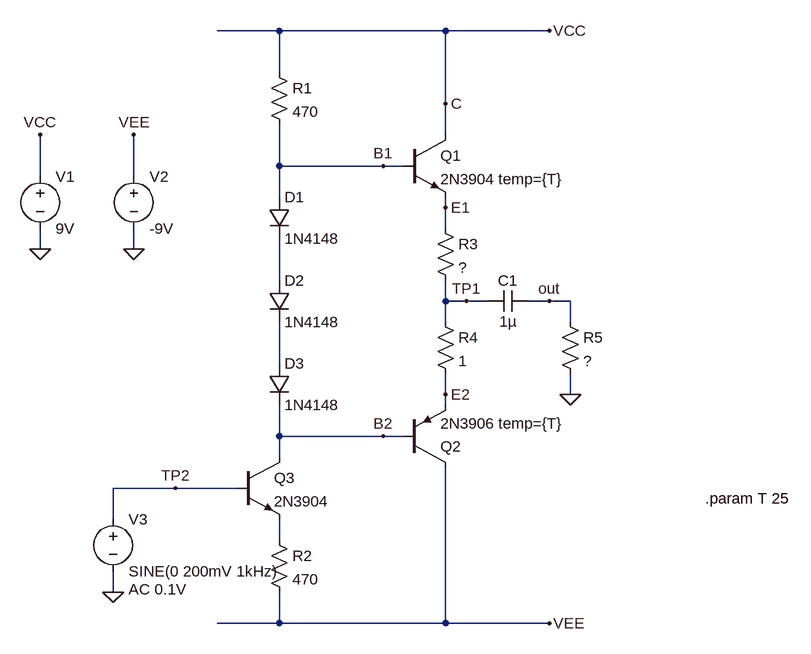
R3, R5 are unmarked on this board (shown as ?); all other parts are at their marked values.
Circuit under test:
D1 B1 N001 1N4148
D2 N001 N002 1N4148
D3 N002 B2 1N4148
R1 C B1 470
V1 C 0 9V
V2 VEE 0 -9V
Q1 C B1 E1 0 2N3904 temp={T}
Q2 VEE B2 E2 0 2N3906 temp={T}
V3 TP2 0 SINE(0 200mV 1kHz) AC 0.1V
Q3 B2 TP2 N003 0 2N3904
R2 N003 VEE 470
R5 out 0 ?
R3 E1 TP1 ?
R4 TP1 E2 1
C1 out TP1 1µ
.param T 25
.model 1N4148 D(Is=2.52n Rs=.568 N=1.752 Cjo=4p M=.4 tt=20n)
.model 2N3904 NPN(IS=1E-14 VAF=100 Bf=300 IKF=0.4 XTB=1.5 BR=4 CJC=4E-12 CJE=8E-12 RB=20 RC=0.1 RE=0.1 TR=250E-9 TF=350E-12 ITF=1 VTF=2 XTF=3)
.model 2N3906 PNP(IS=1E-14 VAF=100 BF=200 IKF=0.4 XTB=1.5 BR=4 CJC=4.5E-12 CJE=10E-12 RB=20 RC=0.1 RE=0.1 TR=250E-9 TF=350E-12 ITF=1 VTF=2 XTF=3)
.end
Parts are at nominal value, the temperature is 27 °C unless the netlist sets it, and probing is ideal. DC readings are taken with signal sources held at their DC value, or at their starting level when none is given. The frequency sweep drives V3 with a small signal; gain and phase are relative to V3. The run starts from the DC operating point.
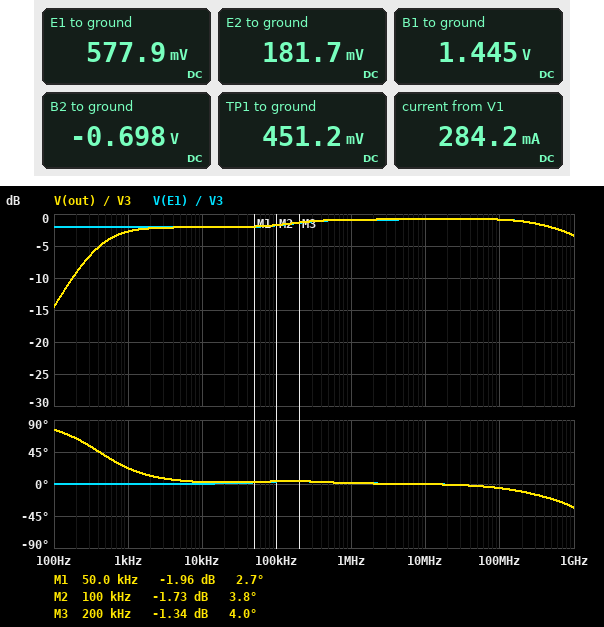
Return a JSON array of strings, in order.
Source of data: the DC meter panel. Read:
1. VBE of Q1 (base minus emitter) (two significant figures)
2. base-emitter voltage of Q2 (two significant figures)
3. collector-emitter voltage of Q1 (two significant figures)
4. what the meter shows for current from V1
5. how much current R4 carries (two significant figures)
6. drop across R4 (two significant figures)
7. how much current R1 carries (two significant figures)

["870 mV", "-880 mV", "8.4 V", "284.2 mA", "270 mA", "270 mV", "16 mA"]
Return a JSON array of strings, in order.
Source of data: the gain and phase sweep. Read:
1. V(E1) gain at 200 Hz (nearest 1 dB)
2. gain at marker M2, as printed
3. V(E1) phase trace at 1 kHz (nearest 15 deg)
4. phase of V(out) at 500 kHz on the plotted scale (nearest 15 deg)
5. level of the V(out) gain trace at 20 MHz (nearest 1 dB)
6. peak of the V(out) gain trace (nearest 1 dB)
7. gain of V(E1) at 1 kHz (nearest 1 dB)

["-2 dB", "-1.73 dB", "0 deg", "0 deg", "-1 dB", "-1 dB", "-2 dB"]
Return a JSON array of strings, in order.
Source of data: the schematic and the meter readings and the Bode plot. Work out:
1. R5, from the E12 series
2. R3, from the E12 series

["390 Ω", "0.47 Ω"]
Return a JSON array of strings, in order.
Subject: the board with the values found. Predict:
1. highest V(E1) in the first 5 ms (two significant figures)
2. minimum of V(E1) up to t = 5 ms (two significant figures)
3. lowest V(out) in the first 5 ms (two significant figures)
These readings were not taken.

["740 mV", "450 mV", "-140 mV"]
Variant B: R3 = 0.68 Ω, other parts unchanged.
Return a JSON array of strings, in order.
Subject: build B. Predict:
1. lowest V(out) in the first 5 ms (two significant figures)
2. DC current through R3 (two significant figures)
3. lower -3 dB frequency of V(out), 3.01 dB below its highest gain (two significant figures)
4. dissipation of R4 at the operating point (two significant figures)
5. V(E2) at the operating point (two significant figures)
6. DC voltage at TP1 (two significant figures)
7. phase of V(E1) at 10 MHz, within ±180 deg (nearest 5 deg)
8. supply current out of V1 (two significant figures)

["-150 mV", "250 mA", "560 Hz", "61 mW", "170 mV", "420 mV", "0 deg", "260 mA"]
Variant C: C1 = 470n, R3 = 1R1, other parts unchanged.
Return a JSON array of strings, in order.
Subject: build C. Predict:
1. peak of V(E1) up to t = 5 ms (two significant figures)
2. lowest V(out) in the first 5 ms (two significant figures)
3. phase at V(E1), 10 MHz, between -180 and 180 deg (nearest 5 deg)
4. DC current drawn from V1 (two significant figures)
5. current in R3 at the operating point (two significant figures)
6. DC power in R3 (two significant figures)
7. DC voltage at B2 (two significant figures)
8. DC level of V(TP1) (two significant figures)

["760 mV", "-120 mV", "0 deg", "230 mA", "210 mA", "50 mW", "-710 mV", "360 mV"]
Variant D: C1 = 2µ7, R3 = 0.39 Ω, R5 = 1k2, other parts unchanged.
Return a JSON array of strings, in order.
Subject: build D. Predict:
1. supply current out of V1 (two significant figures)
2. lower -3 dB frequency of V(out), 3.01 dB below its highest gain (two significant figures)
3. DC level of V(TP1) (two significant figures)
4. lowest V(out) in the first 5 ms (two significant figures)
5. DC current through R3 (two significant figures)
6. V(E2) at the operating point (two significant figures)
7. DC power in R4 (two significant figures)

["290 mA", "72 Hz", "470 mV", "-130 mV", "280 mA", "190 mV", "78 mW"]
